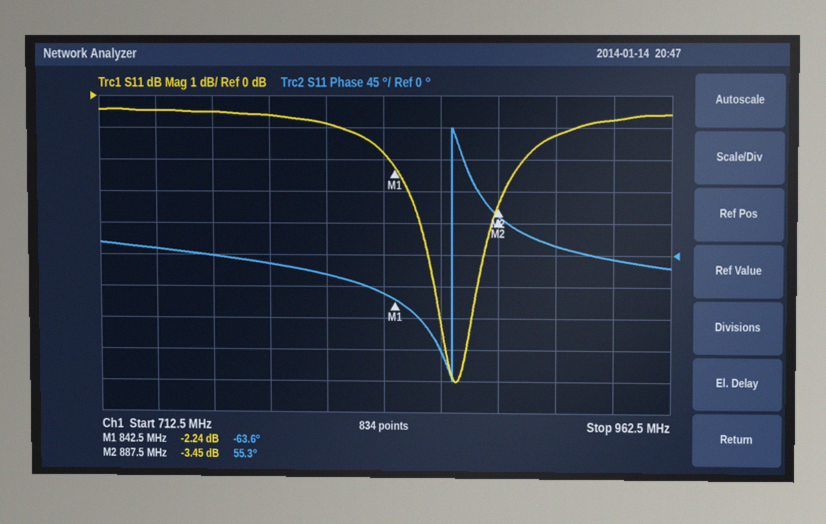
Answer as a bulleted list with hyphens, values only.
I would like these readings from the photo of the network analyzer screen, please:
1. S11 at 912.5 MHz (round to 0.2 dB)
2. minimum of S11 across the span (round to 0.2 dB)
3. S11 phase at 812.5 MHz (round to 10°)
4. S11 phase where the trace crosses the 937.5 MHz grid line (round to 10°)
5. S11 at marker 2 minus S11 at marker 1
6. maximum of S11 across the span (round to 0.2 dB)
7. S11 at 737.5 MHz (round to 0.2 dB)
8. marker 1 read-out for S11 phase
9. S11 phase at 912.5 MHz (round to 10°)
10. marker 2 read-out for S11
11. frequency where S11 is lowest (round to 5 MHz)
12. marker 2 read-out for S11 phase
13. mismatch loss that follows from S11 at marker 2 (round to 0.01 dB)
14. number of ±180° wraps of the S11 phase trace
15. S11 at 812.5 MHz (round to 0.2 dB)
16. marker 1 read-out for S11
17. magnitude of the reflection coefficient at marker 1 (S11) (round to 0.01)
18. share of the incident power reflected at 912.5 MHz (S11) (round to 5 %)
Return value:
- -1.2 dB
- -9.0 dB
- -30°
- -10°
- -1.21 dB
- -0.4 dB
- -0.4 dB
- -63.6°
- 10°
- -3.45 dB
- 870 MHz
- 55.3°
- 2.61 dB
- 1
- -0.8 dB
- -2.24 dB
- 0.77
- 75 %
